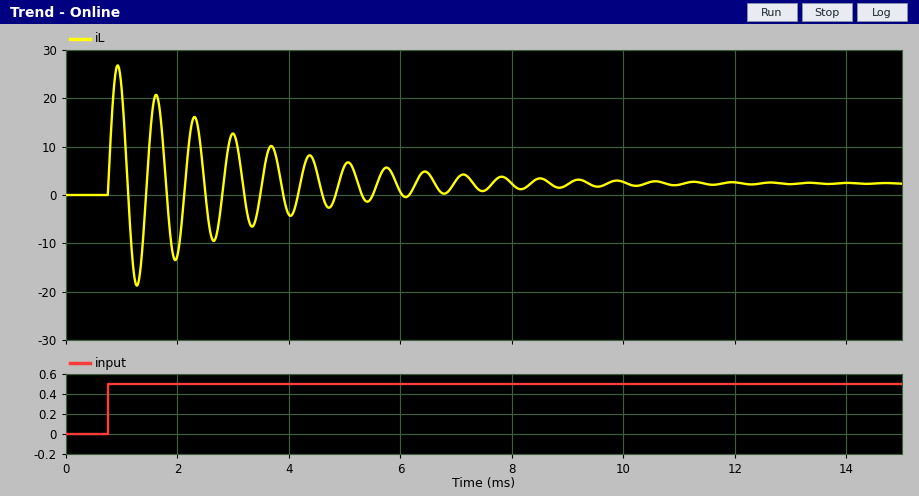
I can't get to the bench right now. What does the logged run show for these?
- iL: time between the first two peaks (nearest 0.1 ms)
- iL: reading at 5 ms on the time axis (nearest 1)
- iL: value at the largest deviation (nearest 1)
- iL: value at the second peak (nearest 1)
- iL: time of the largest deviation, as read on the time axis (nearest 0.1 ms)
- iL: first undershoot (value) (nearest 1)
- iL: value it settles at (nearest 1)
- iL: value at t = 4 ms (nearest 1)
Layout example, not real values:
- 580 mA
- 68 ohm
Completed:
- 0.7 ms
- 6
- 27
- 21
- 0.9 ms
- -19
- 2
- -4
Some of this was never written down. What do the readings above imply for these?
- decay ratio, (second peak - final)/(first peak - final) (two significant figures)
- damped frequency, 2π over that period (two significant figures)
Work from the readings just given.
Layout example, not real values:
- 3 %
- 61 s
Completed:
- 0.76
- 9.0 rad/ms
